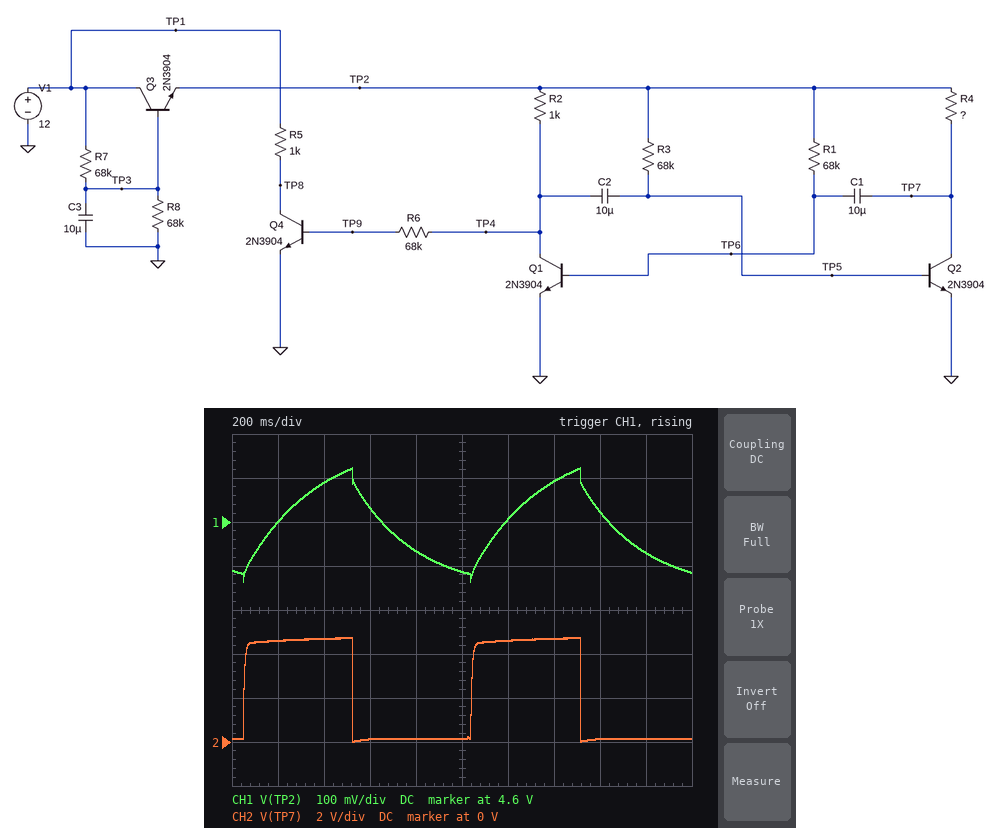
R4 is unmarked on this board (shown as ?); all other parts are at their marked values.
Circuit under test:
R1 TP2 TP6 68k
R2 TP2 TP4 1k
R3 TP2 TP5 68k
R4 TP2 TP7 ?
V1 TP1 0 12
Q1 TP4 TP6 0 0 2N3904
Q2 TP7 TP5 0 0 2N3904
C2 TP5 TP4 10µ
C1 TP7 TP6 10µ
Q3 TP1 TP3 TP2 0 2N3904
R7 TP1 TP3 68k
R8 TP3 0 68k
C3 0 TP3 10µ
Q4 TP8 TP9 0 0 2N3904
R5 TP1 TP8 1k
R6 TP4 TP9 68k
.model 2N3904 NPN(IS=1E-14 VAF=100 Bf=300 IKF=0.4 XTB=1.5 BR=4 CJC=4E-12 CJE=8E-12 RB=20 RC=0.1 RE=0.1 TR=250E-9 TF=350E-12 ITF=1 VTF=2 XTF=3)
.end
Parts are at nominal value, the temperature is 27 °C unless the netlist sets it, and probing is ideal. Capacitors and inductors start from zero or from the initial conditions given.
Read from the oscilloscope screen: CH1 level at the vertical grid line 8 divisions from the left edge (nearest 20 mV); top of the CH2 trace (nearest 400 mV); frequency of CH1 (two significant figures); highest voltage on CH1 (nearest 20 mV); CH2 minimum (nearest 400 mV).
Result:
4.62 V
4.8 V
1.0 Hz
4.72 V
0 V
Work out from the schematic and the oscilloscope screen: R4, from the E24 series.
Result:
560 Ω
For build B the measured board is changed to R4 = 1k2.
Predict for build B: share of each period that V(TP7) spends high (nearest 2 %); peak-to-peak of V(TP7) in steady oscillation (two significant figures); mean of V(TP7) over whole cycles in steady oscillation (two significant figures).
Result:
50 %
4.8 V
2.4 V
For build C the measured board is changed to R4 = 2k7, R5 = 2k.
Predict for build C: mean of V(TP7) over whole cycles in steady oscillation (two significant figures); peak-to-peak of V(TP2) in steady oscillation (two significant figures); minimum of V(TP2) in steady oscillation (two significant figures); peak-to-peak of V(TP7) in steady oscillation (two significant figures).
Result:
2.4 V
230 mV
4.8 V
4.9 V
